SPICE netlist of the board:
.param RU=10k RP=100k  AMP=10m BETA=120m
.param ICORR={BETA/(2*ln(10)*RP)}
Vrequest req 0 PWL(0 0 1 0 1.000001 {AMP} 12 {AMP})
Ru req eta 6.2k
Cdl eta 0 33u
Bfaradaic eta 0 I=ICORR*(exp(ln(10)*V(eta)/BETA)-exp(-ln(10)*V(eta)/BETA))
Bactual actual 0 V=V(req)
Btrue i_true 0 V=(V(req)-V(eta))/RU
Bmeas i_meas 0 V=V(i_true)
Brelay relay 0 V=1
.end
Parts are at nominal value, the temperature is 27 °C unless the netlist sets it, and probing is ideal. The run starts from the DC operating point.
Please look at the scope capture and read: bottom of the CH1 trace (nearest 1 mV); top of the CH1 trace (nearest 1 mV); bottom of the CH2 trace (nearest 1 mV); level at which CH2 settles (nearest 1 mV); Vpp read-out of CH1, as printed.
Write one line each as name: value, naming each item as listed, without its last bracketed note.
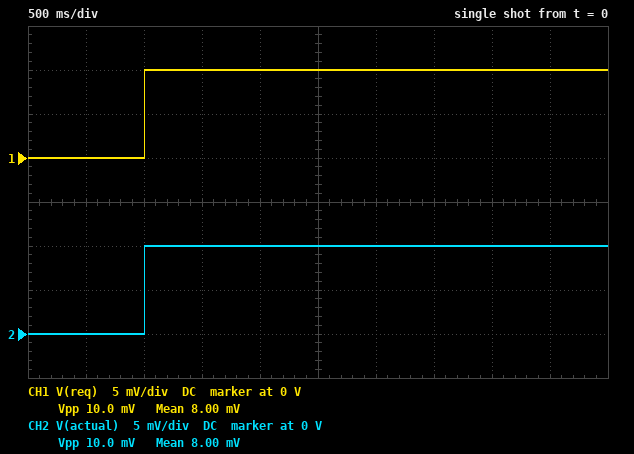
bottom of the CH1 trace: 0 V
top of the CH1 trace: 10 mV
bottom of the CH2 trace: 0 V
level at which CH2 settles: 10 mV
Vpp read-out of CH1, as printed: 10.0 mV
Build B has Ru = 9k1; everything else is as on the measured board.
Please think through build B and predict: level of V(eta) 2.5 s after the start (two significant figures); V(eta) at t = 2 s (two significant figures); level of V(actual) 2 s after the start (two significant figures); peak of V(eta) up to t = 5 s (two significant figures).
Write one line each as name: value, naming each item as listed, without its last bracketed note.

level of V(eta) 2.5 s after the start: 9.1 mV
V(eta) at t = 2 s: 8.9 mV
level of V(actual) 2 s after the start: 10 mV
peak of V(eta) up to t = 5 s: 9.2 mV
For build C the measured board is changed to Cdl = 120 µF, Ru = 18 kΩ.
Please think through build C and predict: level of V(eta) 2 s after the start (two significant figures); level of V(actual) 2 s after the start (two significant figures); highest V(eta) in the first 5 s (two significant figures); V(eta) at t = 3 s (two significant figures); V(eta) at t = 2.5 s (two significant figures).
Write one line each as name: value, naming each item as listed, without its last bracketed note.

level of V(eta) 2 s after the start: 3.6 mV
level of V(actual) 2 s after the start: 10 mV
highest V(eta) in the first 5 s: 7.5 mV
V(eta) at t = 3 s: 5.6 mV
V(eta) at t = 2.5 s: 4.7 mV
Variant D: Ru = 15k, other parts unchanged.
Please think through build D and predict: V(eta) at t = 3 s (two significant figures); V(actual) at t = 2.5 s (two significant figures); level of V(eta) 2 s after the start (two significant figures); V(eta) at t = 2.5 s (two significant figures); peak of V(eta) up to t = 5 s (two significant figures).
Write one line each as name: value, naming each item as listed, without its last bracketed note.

V(eta) at t = 3 s: 8.6 mV
V(actual) at t = 2.5 s: 10 mV
level of V(eta) 2 s after the start: 7.8 mV
V(eta) at t = 2.5 s: 8.4 mV
peak of V(eta) up to t = 5 s: 8.7 mV
